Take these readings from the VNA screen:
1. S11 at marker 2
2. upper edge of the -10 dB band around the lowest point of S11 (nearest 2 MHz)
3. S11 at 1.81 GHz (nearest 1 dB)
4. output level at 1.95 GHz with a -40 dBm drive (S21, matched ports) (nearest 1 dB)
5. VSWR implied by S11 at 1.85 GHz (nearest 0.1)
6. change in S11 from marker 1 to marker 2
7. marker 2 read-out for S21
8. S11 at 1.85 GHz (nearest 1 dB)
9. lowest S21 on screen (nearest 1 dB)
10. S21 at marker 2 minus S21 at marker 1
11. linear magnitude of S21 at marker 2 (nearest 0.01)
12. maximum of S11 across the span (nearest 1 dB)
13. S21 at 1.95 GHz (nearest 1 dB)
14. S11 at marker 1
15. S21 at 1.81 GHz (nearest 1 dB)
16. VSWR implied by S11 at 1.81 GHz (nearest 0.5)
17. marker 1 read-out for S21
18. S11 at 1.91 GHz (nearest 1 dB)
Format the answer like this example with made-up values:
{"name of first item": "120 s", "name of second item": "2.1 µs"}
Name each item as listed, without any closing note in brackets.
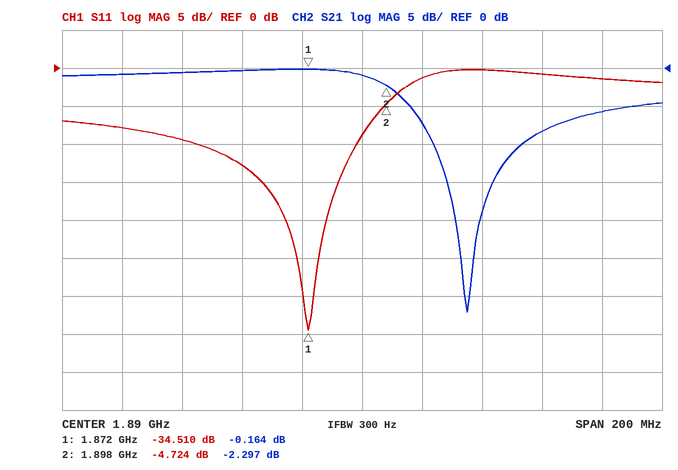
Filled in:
{"S11 at marker 2": "-4.724 dB", "upper edge of the -10 dB band around the lowest point of S11": "1.888 GHz", "S11 at 1.81 GHz": "-8 dB", "output level at 1.95 GHz with a -40 dBm drive (S21, matched ports)": "-48 dBm", "VSWR implied by S11 at 1.85 GHz": "1.6", "change in S11 from marker 1 to marker 2": "29.786 dB", "marker 2 read-out for S21": "-2.297 dB", "S11 at 1.85 GHz": "-13 dB", "lowest S21 on screen": "-32 dB", "S21 at marker 2 minus S21 at marker 1": "-2.133 dB", "linear magnitude of S21 at marker 2": "0.77", "maximum of S11 across the span": "0 dB", "S21 at 1.95 GHz": "-8 dB", "S11 at marker 1": "-34.510 dB", "S21 at 1.81 GHz": "-1 dB", "VSWR implied by S11 at 1.81 GHz": "2.5", "marker 1 read-out for S21": "-0.164 dB", "S11 at 1.91 GHz": "-1 dB"}
